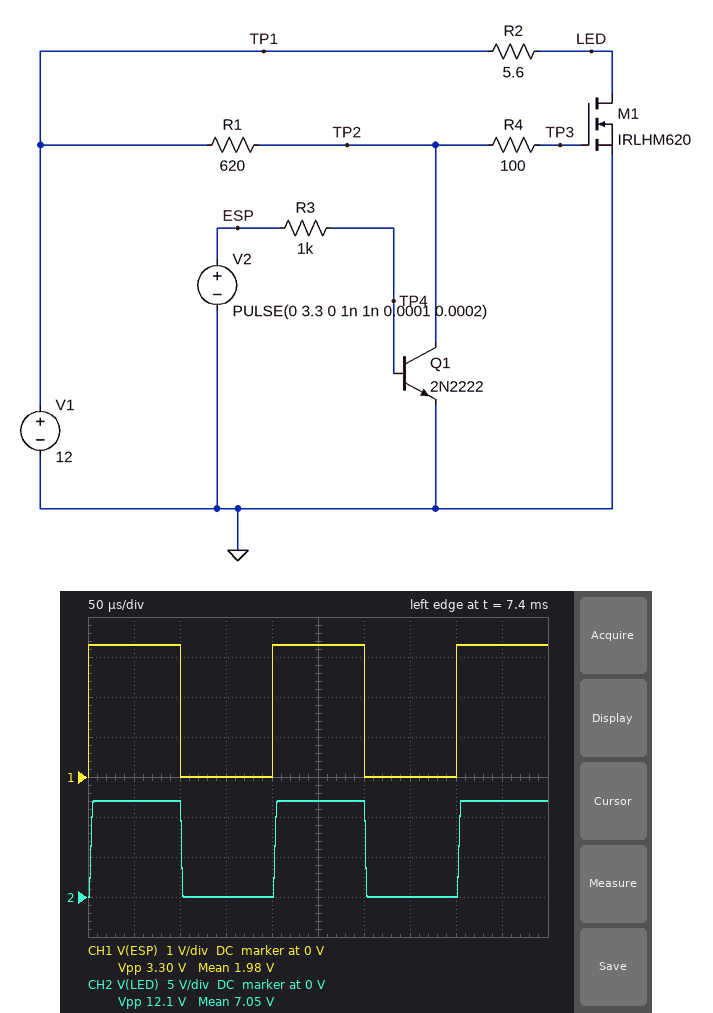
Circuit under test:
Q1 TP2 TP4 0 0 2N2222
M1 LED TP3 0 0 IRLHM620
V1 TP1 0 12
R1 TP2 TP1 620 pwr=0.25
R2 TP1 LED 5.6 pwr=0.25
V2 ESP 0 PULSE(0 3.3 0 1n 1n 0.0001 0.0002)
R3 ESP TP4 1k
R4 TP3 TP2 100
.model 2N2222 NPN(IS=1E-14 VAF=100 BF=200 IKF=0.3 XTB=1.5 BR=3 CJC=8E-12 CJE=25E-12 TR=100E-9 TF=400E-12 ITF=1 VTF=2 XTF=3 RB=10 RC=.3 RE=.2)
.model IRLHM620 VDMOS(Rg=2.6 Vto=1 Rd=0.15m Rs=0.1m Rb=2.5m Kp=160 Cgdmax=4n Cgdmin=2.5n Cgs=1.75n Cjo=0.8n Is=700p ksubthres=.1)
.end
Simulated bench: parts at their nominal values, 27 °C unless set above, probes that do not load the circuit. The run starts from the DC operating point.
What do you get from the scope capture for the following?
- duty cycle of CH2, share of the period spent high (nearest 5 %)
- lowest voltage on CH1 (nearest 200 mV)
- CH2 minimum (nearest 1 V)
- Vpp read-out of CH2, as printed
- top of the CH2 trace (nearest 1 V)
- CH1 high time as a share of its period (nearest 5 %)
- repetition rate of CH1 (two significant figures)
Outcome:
50 %
0 V
0 V
12.1 V
12 V
50 %
5.0 kHz
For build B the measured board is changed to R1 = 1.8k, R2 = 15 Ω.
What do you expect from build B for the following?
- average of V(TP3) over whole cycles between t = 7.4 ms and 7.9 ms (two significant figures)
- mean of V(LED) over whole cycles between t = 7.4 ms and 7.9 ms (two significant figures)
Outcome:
5.1 V
6.0 V
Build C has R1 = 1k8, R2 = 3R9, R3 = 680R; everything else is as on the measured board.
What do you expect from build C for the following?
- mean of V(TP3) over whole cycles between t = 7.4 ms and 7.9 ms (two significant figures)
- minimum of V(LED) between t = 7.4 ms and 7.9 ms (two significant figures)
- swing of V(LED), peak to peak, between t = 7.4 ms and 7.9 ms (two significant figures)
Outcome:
5.1 V
2.5 mV
12 V
